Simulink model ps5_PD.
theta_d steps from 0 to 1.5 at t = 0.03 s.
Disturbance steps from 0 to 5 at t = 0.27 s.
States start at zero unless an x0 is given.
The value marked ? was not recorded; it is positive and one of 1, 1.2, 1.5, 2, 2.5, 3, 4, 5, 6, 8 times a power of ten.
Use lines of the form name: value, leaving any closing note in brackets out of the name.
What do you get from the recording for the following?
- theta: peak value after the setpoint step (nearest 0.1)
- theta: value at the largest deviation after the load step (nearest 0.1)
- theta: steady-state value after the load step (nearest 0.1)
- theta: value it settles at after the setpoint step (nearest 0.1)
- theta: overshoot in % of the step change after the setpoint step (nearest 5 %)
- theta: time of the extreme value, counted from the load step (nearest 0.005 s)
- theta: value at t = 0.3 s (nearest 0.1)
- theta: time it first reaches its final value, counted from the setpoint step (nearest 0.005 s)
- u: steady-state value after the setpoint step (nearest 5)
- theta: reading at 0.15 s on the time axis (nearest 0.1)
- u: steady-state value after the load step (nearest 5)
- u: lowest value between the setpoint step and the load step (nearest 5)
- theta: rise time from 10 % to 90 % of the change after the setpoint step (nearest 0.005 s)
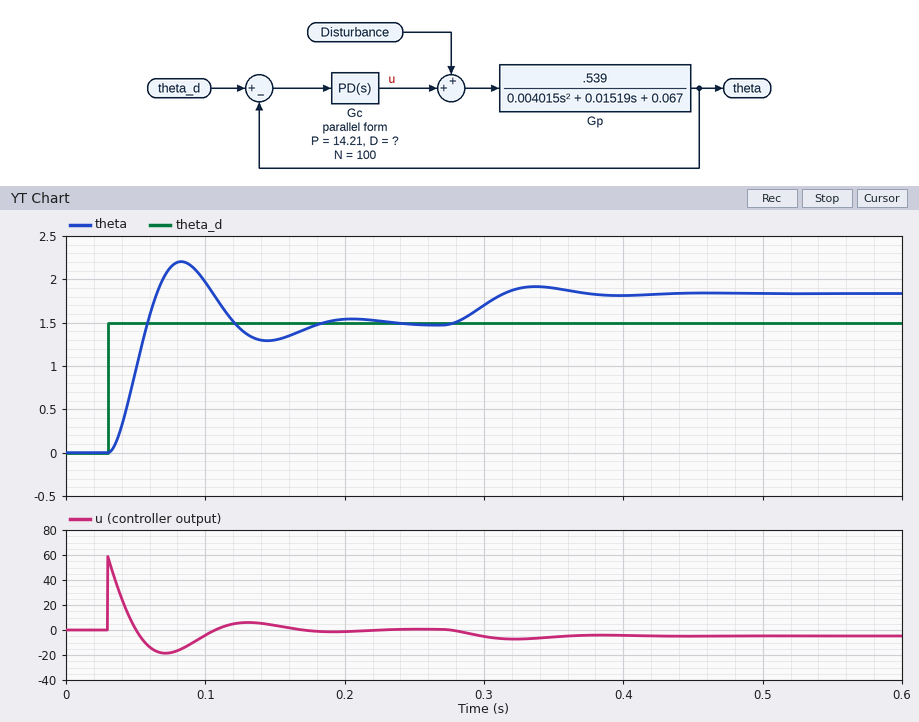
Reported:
theta: peak value after the setpoint step: 2.2
theta: value at the largest deviation after the load step: 1.9
theta: steady-state value after the load step: 1.8
theta: value it settles at after the setpoint step: 1.5
theta: overshoot in % of the step change after the setpoint step: 50 %
theta: time of the extreme value, counted from the load step: 0.065 s
theta: value at t = 0.3 s: 1.7
theta: time it first reaches its final value, counted from the setpoint step: 0.030 s
u: steady-state value after the setpoint step: 0
theta: reading at 0.15 s on the time axis: 1.3
u: steady-state value after the load step: -5
u: lowest value between the setpoint step and the load step: -20
theta: rise time from 10 % to 90 % of the change after the setpoint step: 0.020 s
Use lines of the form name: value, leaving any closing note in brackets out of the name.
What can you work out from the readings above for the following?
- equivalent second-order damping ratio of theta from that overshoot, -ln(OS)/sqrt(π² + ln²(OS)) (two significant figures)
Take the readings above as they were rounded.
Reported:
equivalent second-order damping ratio of theta from that overshoot, -ln(OS)/sqrt(π² + ln²(OS)): 0.22
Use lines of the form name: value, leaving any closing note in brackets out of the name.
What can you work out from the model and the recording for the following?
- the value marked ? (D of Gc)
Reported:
the value marked ?: 0.25
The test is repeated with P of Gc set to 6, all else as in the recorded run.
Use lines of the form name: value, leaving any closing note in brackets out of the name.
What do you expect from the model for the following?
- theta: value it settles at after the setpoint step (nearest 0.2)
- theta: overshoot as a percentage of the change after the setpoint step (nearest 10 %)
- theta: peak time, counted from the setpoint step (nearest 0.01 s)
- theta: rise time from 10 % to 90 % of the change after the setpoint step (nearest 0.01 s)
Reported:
theta: value it settles at after the setpoint step: 1.4
theta: overshoot as a percentage of the change after the setpoint step: 30 %
theta: peak time, counted from the setpoint step: 0.07 s
theta: rise time from 10 % to 90 % of the change after the setpoint step: 0.03 s
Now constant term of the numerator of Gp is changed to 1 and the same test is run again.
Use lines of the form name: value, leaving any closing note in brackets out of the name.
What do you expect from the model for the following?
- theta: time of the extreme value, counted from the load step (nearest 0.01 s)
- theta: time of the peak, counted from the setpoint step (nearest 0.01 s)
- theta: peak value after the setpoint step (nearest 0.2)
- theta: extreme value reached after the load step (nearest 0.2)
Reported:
theta: time of the extreme value, counted from the load step: 0.05 s
theta: time of the peak, counted from the setpoint step: 0.04 s
theta: peak value after the setpoint step: 2.2
theta: extreme value reached after the load step: 1.8
